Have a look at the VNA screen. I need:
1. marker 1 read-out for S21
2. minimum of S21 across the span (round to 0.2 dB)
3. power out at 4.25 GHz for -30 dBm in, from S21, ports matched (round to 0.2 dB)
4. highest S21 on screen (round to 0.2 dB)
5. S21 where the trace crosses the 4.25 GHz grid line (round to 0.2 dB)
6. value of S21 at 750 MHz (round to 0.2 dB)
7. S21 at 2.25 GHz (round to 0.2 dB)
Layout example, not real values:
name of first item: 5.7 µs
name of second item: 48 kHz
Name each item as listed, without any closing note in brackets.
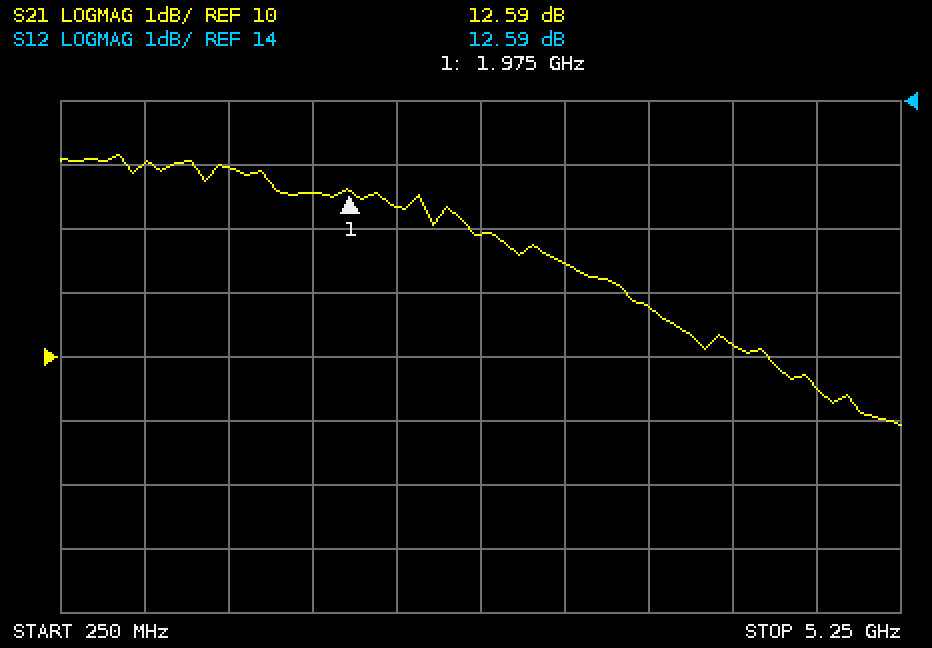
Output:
marker 1 read-out for S21: 12.59 dB
minimum of S21 across the span: 9.0 dB
power out at 4.25 GHz for -30 dBm in, from S21, ports matched: -19.8 dBm
highest S21 on screen: 13.2 dB
S21 where the trace crosses the 4.25 GHz grid line: 10.2 dB
value of S21 at 750 MHz: 13.0 dB
S21 at 2.25 GHz: 12.4 dB
